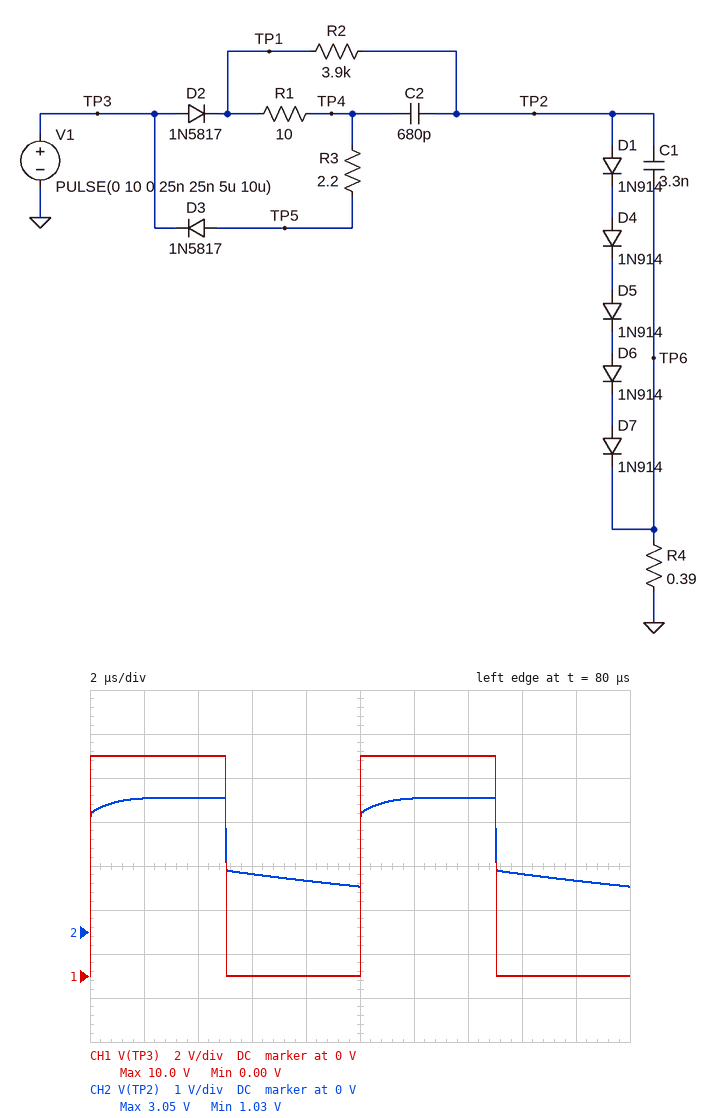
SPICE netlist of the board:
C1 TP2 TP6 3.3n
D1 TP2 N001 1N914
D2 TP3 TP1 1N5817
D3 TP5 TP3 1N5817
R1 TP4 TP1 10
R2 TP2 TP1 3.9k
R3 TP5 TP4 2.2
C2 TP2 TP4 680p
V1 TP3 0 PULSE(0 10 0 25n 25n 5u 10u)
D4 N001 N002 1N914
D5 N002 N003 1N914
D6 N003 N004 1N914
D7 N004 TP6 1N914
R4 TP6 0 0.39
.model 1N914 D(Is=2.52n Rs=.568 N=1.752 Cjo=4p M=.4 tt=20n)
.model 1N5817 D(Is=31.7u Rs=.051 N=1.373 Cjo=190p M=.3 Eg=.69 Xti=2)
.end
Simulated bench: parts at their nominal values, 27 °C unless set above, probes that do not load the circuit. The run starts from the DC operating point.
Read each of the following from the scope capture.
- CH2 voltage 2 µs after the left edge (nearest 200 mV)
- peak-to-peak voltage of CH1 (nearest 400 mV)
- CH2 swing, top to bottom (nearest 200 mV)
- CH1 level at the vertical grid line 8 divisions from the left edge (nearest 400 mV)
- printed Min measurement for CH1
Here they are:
3.0 V
10.0 V
2.0 V
0 V
0.00 V
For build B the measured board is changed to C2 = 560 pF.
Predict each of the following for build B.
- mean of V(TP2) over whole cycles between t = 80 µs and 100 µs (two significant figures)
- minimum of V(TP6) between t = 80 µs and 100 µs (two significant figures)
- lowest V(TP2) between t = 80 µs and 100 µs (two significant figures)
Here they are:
2.2 V
-75 mV
1.2 V
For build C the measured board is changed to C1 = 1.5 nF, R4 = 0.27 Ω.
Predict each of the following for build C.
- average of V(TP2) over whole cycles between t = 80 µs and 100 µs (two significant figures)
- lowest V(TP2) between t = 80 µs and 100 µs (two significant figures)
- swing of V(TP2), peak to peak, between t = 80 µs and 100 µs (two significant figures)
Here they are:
1.5 V
3.9 mV
3.1 V
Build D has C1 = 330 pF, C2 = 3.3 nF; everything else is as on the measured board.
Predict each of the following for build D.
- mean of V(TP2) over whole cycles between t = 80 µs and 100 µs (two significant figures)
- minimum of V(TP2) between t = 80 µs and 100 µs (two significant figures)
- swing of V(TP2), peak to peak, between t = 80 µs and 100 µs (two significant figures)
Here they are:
-920 mV
-5.8 V
9.7 V
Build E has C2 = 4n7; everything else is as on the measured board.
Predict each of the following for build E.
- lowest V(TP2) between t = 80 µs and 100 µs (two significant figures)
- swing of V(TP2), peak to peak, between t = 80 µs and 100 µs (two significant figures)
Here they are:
-2.7 V
6.0 V
